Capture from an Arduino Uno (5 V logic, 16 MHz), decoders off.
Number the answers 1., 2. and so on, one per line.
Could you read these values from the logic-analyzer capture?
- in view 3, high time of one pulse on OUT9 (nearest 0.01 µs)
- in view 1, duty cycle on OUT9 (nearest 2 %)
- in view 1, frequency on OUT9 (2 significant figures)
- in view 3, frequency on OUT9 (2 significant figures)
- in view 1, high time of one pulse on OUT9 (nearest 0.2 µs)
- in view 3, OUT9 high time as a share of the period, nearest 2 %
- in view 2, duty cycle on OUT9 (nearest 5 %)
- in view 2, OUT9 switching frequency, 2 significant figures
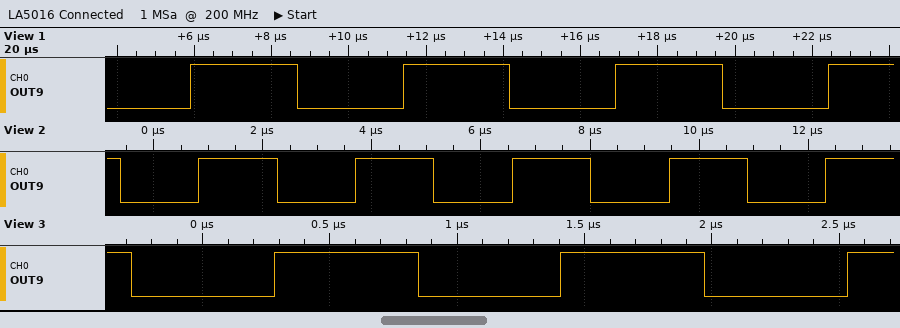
1. 0.56 µs
2. 50 %
3. 180 kHz
4. 890 kHz
5. 2.8 µs
6. 50 %
7. 50 %
8. 350 kHz
